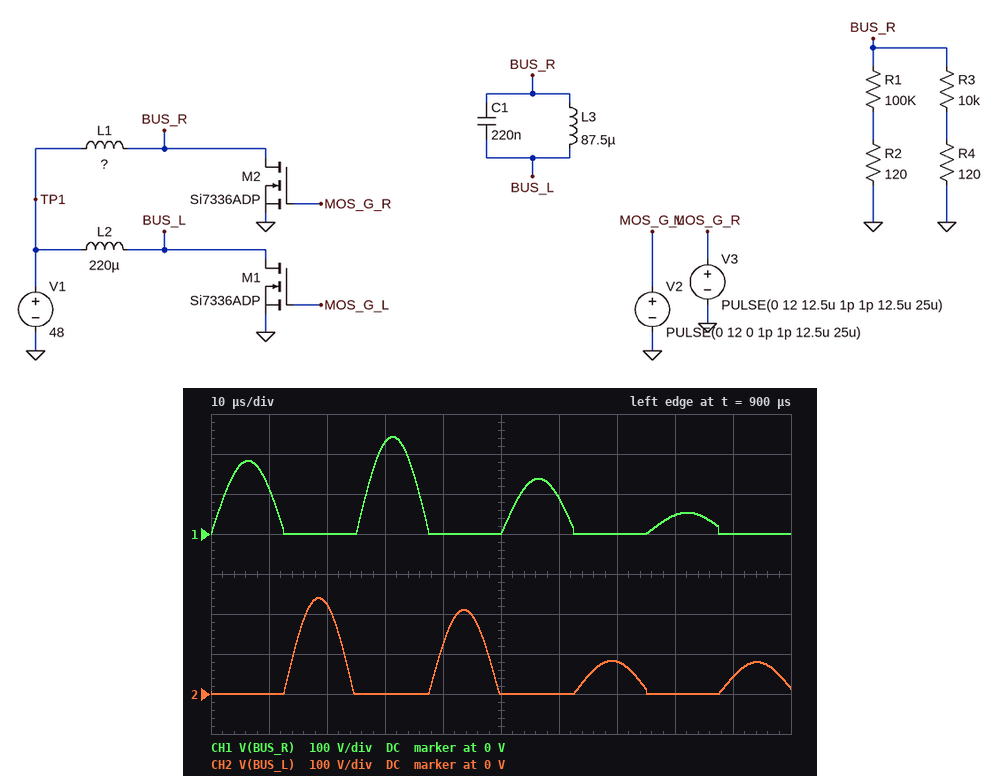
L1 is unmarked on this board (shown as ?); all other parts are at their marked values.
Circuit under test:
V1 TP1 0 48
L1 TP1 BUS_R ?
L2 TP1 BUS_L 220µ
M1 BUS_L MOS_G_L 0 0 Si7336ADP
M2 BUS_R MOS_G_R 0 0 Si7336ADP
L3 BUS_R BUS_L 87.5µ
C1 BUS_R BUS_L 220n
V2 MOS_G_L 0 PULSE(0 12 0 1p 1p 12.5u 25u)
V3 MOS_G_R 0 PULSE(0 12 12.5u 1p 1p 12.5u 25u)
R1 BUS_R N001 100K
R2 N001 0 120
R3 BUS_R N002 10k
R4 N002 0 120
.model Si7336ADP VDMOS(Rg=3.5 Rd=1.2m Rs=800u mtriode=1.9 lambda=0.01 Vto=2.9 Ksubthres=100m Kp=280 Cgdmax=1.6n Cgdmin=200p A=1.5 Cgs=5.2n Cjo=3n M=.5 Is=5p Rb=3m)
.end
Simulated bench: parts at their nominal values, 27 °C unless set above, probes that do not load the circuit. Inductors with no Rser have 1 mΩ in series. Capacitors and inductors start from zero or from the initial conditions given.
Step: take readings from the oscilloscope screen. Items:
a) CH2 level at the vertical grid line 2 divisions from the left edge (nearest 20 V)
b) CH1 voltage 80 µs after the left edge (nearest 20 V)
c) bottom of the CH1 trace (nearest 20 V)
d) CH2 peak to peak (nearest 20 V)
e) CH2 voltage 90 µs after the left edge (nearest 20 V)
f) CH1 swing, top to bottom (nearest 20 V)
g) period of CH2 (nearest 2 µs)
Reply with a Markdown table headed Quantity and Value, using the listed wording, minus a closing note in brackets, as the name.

| Quantity | Value |
|---|---|
| CH2 level at the vertical grid line 2 divisions from the left edge | 220 V |
| CH1 voltage 80 µs after the left edge | 40 V |
| bottom of the CH1 trace | 0 V |
| CH2 peak to peak | 240 V |
| CH2 voltage 90 µs after the left edge | 40 V |
| CH1 swing, top to bottom | 240 V |
| period of CH2 | 26 µs |
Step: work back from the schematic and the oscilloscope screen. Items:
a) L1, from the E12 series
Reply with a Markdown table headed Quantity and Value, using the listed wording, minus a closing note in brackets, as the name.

| Quantity | Value |
|---|---|
| L1, from the E12 series | 330 µH |
